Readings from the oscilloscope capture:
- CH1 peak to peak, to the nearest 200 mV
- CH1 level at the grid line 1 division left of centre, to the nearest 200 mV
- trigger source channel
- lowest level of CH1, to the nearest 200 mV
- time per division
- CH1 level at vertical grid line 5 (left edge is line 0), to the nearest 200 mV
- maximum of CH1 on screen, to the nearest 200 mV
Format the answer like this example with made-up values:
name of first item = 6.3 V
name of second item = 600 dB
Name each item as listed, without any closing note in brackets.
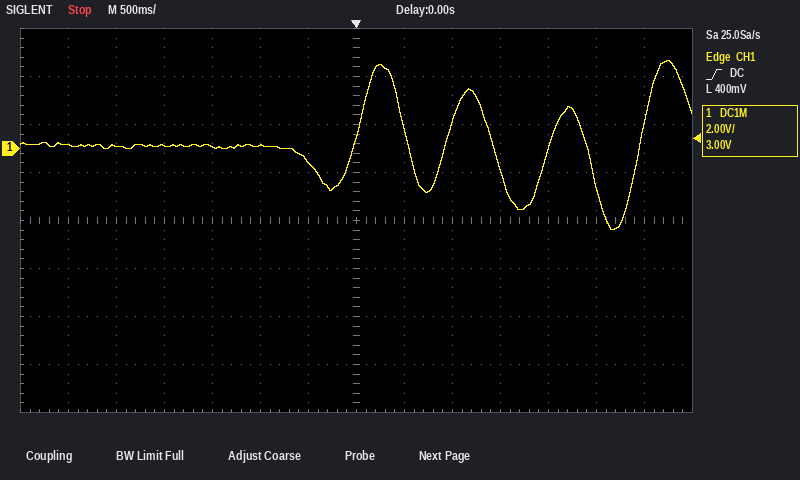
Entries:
CH1 peak to peak, to the nearest 200 mV = 7.0 V
CH1 level at the grid line 1 division left of centre, to the nearest 200 mV = -600 mV
trigger source channel = CH1
lowest level of CH1, to the nearest 200 mV = -3.4 V
time per division = 500 ms
CH1 level at vertical grid line 5 (left edge is line 0), to the nearest 200 mV = 200 mV
maximum of CH1 on screen, to the nearest 200 mV = 3.6 V
